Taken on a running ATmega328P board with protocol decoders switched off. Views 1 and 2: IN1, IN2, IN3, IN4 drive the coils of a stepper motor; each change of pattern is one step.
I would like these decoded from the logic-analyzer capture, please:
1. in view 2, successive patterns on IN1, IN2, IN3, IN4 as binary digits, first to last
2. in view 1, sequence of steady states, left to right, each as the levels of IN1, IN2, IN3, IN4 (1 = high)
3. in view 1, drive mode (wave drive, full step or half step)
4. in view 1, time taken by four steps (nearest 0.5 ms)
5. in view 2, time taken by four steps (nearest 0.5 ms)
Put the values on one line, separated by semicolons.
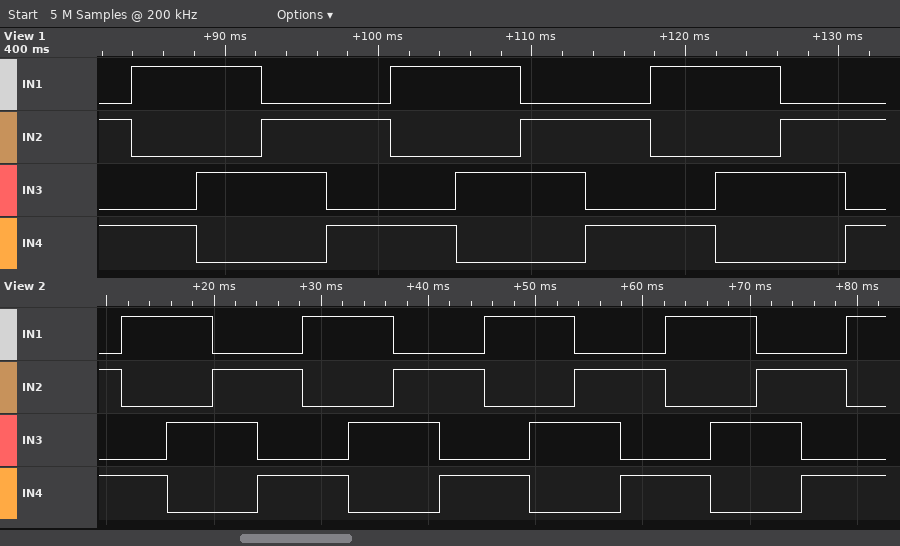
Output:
0101 1001 1010 0110 0101 1001 1010 0110 0101 1001 1010 0110 0101 1001 1010 0110 0101 1001; 0101 1001 1010 0110 0101 1001 1010 0110 0101 1001 1010 0110 0101; full step; 17.0 ms; 17.0 ms
